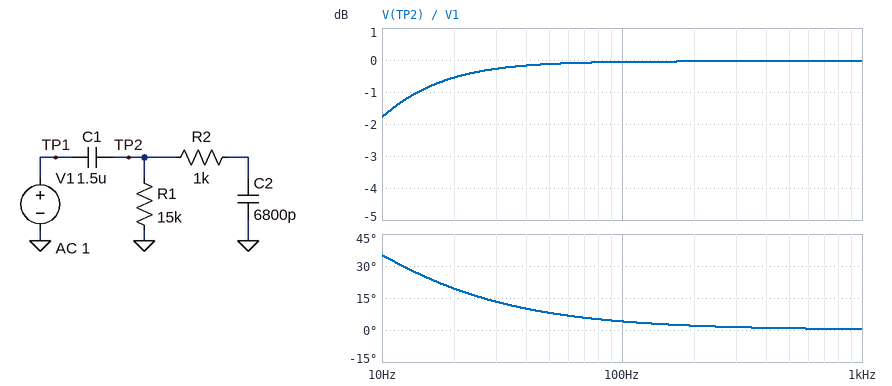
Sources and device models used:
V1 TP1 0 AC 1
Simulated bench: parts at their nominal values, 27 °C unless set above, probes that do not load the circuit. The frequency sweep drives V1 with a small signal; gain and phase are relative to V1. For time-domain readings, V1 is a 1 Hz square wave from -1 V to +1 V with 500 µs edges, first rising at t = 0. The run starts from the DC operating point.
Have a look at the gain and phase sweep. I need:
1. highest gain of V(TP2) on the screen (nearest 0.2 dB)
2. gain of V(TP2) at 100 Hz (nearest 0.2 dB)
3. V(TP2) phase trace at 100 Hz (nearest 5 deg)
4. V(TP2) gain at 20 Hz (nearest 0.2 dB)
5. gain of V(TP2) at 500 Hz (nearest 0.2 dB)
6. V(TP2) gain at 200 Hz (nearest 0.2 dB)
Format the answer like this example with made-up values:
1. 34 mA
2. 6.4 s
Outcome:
1. 0 dB
2. 0 dB
3. 5 deg
4. -0.6 dB
5. 0 dB
6. 0 dB
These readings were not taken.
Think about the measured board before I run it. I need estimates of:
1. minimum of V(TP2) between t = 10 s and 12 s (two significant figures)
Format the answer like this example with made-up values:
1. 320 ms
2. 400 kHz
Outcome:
1. -2.0 V
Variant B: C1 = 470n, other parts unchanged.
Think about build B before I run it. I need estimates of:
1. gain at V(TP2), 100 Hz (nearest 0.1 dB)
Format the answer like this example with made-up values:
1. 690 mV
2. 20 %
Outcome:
1. -0.3 dB
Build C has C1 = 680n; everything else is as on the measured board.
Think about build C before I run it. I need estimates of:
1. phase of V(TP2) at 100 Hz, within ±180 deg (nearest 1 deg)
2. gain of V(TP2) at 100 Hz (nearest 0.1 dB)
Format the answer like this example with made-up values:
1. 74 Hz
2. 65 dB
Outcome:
1. 9 deg
2. -0.2 dB
